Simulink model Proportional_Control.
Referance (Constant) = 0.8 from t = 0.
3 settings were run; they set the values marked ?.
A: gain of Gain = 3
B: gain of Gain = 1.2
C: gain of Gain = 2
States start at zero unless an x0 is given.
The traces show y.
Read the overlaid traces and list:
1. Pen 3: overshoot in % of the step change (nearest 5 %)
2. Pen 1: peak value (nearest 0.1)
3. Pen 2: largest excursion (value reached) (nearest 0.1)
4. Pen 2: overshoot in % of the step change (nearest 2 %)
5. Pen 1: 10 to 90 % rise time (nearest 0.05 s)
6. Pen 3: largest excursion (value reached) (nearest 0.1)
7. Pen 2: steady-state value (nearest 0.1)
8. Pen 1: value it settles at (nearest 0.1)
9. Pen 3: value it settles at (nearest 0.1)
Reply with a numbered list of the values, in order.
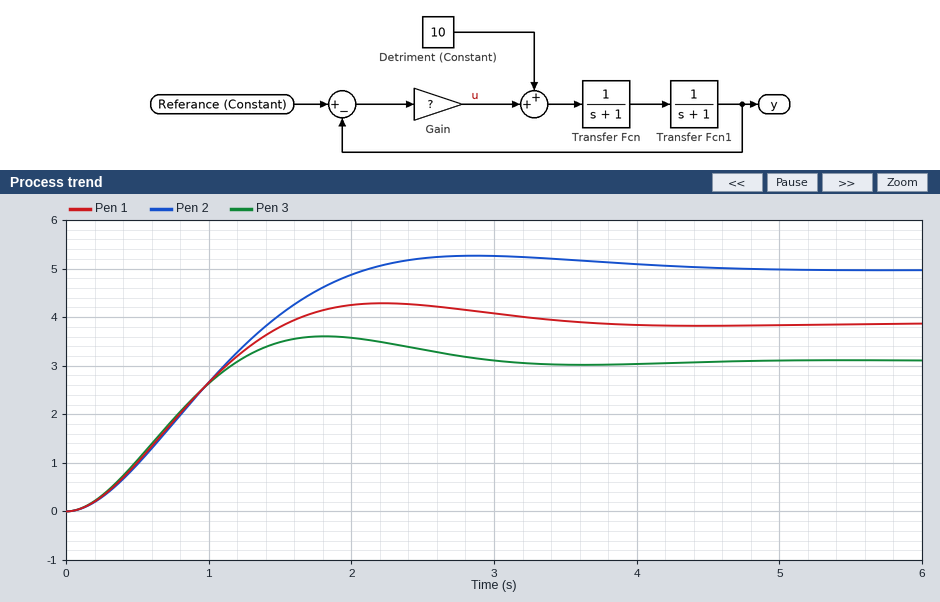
1. 15 %
2. 4.3
3. 5.3
4. 6 %
5. 1.05 s
6. 3.6
7. 5.0
8. 3.9
9. 3.1
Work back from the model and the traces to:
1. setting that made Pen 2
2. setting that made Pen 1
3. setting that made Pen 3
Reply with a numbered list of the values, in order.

1. B
2. C
3. A
